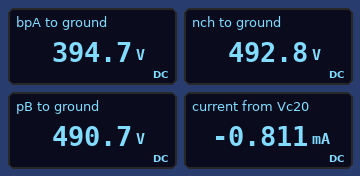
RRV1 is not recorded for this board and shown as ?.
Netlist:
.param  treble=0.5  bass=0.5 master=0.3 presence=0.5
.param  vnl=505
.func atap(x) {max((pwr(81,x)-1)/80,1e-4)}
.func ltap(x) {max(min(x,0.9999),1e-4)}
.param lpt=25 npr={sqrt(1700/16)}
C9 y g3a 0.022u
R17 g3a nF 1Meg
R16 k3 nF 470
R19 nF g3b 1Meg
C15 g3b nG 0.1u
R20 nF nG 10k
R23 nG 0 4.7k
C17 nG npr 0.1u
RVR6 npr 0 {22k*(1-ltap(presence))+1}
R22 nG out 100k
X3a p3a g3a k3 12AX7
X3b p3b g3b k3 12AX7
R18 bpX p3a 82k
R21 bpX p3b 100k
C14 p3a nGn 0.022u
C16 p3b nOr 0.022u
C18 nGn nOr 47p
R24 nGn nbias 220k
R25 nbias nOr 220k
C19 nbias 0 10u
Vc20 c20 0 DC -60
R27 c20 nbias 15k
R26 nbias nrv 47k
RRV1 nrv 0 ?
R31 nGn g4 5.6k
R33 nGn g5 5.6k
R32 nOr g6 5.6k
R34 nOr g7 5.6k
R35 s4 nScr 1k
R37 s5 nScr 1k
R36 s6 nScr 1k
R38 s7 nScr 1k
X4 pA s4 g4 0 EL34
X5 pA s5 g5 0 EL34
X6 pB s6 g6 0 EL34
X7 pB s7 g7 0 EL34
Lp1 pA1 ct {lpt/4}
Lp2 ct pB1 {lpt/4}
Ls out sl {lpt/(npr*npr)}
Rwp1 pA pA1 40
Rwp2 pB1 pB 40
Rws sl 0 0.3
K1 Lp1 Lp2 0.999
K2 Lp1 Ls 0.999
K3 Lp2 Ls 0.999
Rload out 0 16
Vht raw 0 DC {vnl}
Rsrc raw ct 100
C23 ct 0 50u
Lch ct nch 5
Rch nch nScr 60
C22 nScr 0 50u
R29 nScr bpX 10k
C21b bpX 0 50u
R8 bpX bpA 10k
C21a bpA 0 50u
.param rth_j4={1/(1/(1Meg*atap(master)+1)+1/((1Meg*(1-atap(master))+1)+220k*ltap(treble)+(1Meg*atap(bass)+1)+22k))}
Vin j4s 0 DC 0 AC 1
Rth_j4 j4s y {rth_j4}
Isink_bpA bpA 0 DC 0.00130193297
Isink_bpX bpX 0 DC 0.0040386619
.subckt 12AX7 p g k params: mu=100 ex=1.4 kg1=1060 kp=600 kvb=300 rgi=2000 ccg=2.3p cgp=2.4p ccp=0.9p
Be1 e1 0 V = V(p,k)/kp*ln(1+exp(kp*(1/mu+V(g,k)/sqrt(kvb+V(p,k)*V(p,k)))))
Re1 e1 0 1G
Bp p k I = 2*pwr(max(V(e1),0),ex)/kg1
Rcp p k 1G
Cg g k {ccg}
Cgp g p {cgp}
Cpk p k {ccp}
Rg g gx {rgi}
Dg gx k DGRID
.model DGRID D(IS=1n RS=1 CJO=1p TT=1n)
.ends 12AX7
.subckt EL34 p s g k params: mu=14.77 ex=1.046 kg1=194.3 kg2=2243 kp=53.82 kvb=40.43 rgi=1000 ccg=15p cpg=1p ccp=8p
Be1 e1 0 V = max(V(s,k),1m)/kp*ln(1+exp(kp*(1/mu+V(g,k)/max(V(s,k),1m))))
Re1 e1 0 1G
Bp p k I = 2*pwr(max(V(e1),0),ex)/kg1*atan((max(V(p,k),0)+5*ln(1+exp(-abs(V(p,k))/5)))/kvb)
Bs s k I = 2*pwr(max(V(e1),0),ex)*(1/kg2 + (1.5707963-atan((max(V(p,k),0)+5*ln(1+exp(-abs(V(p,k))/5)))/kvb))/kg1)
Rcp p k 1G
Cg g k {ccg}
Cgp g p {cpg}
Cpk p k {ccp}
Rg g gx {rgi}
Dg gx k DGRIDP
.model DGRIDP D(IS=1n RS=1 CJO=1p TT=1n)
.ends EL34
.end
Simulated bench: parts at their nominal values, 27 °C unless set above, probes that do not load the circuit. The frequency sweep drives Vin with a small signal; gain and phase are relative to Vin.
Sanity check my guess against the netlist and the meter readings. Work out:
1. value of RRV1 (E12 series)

12 kΩ
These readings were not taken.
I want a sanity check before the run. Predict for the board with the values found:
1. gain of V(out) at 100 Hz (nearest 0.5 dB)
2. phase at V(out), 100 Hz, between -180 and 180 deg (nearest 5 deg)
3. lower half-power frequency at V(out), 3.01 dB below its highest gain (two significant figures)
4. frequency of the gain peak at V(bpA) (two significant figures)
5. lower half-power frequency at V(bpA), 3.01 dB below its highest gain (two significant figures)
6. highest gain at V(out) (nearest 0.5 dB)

21.0 dB
20 deg
19 Hz
180 mHz
74 mHz
22.0 dB
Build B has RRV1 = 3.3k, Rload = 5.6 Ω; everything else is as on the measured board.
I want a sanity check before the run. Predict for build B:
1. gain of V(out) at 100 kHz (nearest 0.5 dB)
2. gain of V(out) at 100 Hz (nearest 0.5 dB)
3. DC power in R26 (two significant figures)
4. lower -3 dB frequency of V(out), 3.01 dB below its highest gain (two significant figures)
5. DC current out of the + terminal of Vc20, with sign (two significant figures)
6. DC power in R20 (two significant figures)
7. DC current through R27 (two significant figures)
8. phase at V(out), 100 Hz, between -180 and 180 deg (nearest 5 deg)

8.5 dB
15.5 dB
40 mW
27 Hz
-920 µA
92 mW
920 µA
20 deg
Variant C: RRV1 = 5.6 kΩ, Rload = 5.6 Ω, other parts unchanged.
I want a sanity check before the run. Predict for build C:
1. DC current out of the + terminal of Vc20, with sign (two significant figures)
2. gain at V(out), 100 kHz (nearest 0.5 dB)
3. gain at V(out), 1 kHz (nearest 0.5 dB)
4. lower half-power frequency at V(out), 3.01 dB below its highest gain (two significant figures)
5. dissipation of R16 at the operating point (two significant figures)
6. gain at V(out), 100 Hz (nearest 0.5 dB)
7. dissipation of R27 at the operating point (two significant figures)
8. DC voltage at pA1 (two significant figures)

-890 µA
8.0 dB
16.0 dB
27 Hz
4.3 mW
15.0 dB
12 mW
490 V
